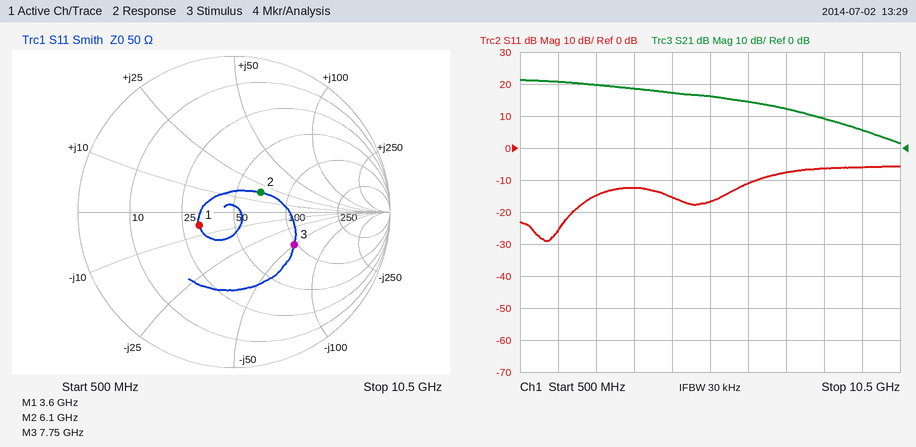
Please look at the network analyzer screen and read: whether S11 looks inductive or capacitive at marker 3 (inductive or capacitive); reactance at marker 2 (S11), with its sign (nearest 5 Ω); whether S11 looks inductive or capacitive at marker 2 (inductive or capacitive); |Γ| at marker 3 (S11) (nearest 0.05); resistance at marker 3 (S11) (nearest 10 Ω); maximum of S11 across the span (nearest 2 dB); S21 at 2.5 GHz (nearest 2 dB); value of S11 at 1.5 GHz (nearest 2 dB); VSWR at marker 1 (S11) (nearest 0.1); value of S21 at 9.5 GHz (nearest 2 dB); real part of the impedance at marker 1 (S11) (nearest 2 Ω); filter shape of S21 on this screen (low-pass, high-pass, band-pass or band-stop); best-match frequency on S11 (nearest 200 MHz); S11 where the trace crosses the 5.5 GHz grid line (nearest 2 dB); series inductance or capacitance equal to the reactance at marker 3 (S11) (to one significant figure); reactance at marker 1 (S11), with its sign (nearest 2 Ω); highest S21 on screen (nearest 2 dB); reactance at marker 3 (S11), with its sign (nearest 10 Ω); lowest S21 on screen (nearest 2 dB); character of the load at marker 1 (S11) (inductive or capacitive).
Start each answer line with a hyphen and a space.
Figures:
- capacitive
- +20 Ω
- inductive
- 0.45
- 100 Ω
- -6 dB
- 20 dB
- -26 dB
- 1.6
- 6 dB
- 32 Ω
- low-pass
- 1.2 GHz
- -16 dB
- 400 fF
- -6 Ω
- 22 dB
- -50 Ω
- 2 dB
- capacitive
